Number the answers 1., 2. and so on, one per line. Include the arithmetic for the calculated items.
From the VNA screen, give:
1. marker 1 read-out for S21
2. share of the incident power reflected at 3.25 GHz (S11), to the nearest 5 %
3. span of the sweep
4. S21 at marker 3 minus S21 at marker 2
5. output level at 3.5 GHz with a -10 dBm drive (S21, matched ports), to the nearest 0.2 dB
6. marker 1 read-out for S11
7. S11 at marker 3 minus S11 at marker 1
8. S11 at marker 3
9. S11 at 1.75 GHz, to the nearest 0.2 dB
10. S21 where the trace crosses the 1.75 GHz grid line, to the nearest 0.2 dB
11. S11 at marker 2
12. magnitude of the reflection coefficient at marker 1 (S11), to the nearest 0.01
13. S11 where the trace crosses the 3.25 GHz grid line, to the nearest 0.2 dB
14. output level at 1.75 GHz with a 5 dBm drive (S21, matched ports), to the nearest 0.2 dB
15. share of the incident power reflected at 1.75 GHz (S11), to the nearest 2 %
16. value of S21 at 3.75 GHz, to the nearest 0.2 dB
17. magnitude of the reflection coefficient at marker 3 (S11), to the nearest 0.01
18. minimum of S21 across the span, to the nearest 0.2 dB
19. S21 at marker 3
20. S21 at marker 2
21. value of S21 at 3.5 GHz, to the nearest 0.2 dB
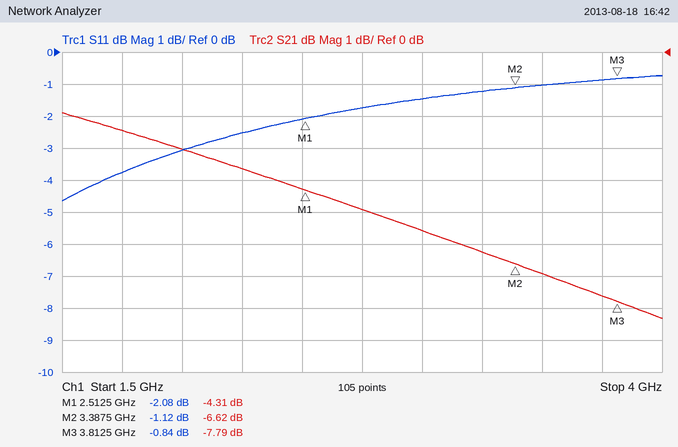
1. -4.31 dB
2. 10^(-1.2/10) ≈ 75.9 %, so 75 % to the nearest 5 %
3. 2.5 GHz
4. -7.79 − (-6.62) = -1.17 dB
5. -10 dBm + (-7.0 dB) = -17.0 dBm
6. -2.08 dB
7. -0.84 − (-2.08) = 1.24 dB
8. -0.84 dB
9. -3.8 dB
10. -2.4 dB
11. -1.12 dB
12. 10^(-2.08/20) ≈ 0.79
13. -1.2 dB
14. 5 dBm + (-2.4 dB) = 2.6 dBm
15. 10^(-3.8/10) ≈ 42 %
16. -7.6 dB
17. 10^(-0.84/20) ≈ 0.91
18. -8.4 dB
19. -7.79 dB
20. -6.62 dB
21. -7.0 dB
